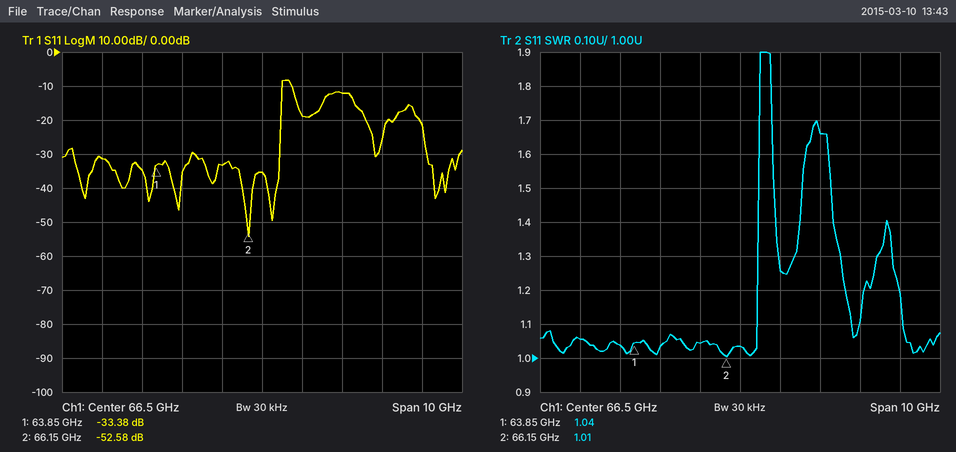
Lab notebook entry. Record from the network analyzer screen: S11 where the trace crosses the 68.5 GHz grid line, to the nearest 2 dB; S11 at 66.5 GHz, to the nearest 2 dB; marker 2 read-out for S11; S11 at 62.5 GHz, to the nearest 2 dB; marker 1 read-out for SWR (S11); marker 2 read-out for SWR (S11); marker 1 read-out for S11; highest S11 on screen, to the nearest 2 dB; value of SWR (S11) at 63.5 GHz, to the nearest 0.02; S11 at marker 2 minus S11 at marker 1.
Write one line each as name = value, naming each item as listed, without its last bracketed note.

S11 where the trace crosses the 68.5 GHz grid line, to the nearest 2 dB = -12 dB
S11 at 66.5 GHz, to the nearest 2 dB = -36 dB
marker 2 read-out for S11 = -52.58 dB
S11 at 62.5 GHz, to the nearest 2 dB = -32 dB
marker 1 read-out for SWR = 1.04
marker 2 read-out for SWR = 1.01
marker 1 read-out for S11 = -33.38 dB
highest S11 on screen, to the nearest 2 dB = -8 dB
value of SWR (S11) at 63.5 GHz, to the nearest 0.02 = 1.04
S11 at marker 2 minus S11 at marker 1 = -19.20 dB
